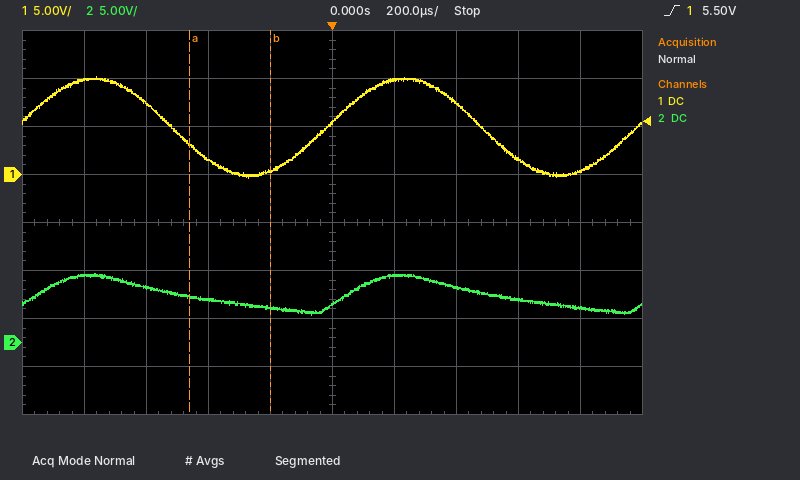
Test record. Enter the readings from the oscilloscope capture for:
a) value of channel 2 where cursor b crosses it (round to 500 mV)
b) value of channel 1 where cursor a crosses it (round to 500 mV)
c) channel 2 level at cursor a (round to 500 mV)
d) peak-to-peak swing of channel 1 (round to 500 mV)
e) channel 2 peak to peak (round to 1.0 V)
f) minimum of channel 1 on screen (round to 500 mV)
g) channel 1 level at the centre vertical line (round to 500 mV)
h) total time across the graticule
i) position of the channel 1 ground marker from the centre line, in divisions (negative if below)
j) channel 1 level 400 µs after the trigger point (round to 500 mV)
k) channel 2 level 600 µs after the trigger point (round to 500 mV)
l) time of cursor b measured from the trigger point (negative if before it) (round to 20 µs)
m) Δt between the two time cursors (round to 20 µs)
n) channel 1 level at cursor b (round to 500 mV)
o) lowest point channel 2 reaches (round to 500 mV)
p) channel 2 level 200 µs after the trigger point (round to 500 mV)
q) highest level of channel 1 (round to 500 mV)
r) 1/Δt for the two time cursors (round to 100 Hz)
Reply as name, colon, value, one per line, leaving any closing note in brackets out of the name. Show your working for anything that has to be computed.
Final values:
value of channel 2 where cursor b crosses it: 3.5 V
value of channel 1 where cursor a crosses it: 3.0 V
channel 2 level at cursor a: 5.0 V
peak-to-peak swing of channel 1: 10.0 V − (-500 mV) = 10.5 V
channel 2 peak to peak: 4.0 V
minimum of channel 1 on screen: -500 mV
channel 1 level at the centre vertical line: 5.5 V
total time across the graticule: 2 ms
position of the channel 1 ground marker from the centre line, in divisions: +1.0 div
channel 1 level 400 µs after the trigger point: 7.5 V
channel 2 level 600 µs after the trigger point: 4.5 V
time of cursor b measured from the trigger point (negative if before it): -200 µs
Δt between the two time cursors: 260 µs
channel 1 level at cursor b: 500 mV
lowest point channel 2 reaches: 3.0 V
channel 2 level 200 µs after the trigger point: 7.0 V
highest level of channel 1: 10.0 V
1/Δt for the two time cursors: 1 / 260 µs ≈ 3.8 kHz
